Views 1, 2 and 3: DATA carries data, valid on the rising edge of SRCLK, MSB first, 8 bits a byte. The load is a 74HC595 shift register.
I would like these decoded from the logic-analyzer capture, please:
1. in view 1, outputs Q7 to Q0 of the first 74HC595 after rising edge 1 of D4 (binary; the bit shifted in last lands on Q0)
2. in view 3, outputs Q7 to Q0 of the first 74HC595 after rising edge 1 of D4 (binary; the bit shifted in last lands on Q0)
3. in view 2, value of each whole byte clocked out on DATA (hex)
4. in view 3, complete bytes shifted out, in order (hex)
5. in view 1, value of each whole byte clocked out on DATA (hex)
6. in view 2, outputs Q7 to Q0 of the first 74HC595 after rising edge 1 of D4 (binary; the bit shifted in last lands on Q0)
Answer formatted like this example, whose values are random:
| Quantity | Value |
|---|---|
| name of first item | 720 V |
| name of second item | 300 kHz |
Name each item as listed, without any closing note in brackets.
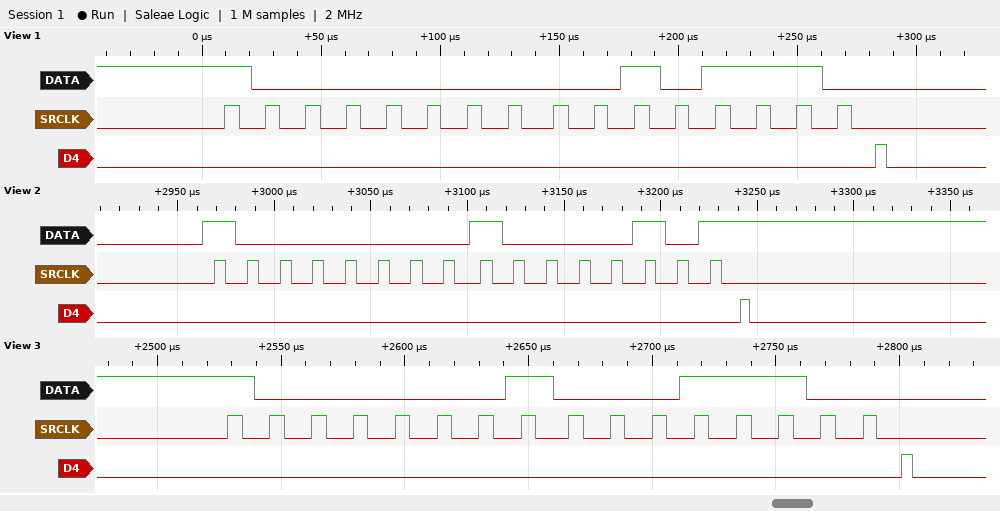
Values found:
| Quantity | Value |
|---|---|
| in view 1, outputs Q7 to Q0 of the first 74HC595 after rising edge 1 of D4 | 00101110 |
| in view 3, outputs Q7 to Q0 of the first 74HC595 after rising edge 1 of D4 | 00011100 |
| in view 2, value of each whole byte clocked out on DATA | 0x80 0x85 |
| in view 3, complete bytes shifted out, in order | 81 1C |
| in view 1, value of each whole byte clocked out on DATA | 80 2E |
| in view 2, outputs Q7 to Q0 of the first 74HC595 after rising edge 1 of D4 | 10000101 |
